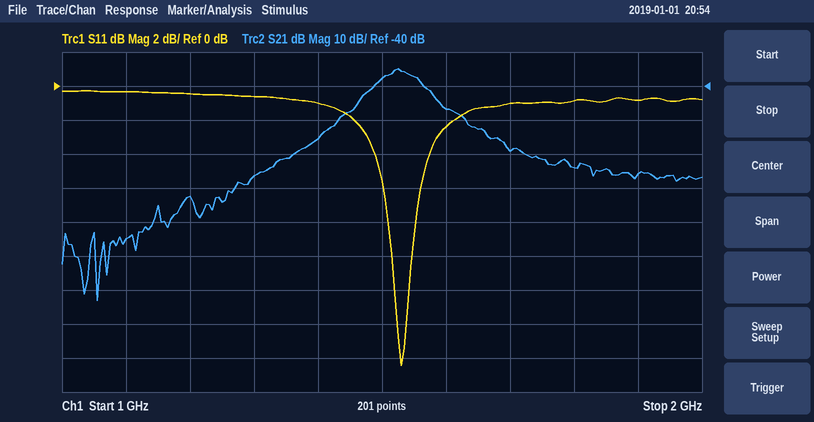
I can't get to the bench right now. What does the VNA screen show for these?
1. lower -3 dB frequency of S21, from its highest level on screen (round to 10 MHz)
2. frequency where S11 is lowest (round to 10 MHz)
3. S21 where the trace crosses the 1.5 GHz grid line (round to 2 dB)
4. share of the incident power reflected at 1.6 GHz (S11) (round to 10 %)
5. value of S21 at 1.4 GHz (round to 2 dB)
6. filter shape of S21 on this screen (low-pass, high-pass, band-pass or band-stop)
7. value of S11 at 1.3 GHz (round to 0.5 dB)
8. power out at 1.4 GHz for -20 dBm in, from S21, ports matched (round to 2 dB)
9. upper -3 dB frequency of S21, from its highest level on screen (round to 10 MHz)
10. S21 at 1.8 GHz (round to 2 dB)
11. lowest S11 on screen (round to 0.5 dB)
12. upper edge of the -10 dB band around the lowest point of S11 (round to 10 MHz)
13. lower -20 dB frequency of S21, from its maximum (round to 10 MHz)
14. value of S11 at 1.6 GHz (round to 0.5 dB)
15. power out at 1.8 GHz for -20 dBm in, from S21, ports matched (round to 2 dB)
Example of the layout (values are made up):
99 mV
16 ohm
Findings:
1.50 GHz
1.53 GHz
-38 dB
60 %
-56 dB
band-pass
-0.5 dB
-76 dBm
1.56 GHz
-64 dB
-16.5 dB
1.55 GHz
1.40 GHz
-2.5 dB
-84 dBm
